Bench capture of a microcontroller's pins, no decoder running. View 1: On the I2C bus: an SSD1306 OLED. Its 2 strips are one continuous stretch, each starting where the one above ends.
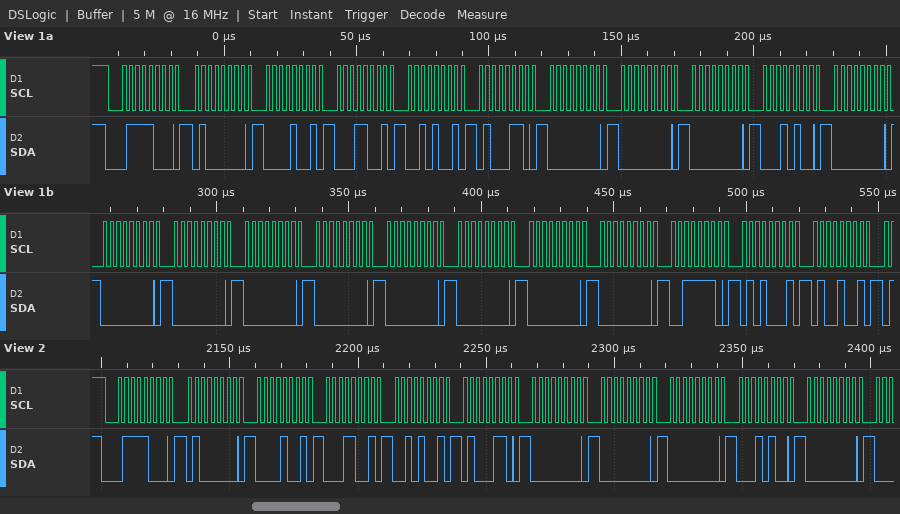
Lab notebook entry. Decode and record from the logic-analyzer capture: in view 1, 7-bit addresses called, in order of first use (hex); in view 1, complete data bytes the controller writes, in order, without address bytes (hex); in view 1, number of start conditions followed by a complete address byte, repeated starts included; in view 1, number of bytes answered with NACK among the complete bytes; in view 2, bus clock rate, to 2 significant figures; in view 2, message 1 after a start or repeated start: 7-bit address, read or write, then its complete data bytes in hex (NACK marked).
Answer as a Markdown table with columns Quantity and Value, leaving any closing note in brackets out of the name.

| Quantity | Value |
|---|---|
| in view 1, 7-bit addresses called, in order of first use | 0x3C |
| in view 1, complete data bytes the controller writes, in order, without address bytes | 40 09 19 29 46 00 00 00 14 00 00 00 00 00 00 00 00 00 3E 51 49 |
| in view 1, number of start conditions followed by a complete address byte, repeated starts included | 1 |
| in view 1, number of bytes answered with NACK among the complete bytes | 0 |
| in view 2, bus clock rate, to 2 significant figures | 400 kHz |
| in view 2, message 1 after a start or repeated start: 7-bit address, read or write, then its complete data bytes in hex | 0x3C write: 40 09 19 29 46 00 00 00 14 00 |
